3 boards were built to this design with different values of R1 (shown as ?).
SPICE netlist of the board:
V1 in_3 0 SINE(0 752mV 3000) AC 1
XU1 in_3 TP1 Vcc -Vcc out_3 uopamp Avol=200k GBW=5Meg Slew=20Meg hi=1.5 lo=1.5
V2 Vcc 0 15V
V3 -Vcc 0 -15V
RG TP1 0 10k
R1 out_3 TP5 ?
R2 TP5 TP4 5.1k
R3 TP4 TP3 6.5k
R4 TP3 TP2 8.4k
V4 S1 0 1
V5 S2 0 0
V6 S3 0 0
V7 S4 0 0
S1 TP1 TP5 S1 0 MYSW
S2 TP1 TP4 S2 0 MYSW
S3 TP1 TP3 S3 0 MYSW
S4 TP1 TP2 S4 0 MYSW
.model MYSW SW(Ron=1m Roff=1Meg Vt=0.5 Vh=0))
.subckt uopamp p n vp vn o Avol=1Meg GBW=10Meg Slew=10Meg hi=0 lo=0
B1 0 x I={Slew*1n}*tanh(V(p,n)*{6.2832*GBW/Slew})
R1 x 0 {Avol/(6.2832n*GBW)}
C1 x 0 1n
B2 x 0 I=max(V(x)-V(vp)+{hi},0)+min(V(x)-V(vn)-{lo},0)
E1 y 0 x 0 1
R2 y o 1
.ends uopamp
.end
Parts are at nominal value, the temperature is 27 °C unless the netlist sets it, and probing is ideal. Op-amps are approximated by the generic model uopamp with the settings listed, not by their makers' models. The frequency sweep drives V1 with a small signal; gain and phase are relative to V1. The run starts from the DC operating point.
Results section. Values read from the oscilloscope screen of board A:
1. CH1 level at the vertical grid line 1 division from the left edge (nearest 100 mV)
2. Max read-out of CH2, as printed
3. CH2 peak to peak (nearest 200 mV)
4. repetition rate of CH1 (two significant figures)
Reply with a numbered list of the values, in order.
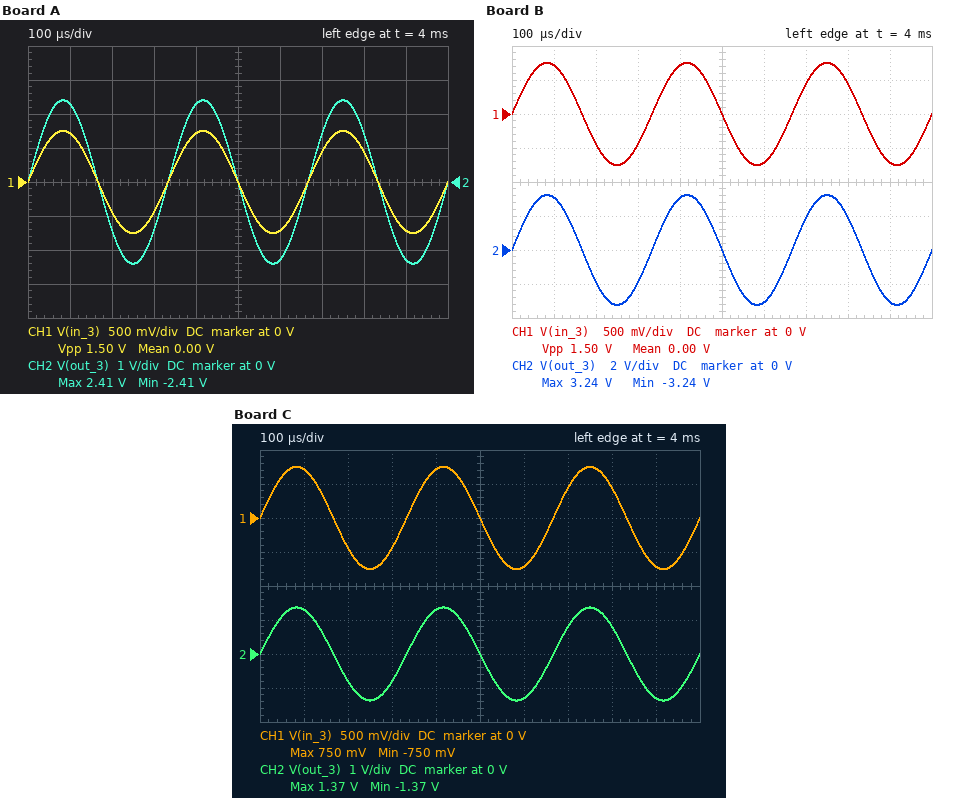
1. 700 mV
2. 2.41 V
3. 4.8 V
4. 3.0 kHz
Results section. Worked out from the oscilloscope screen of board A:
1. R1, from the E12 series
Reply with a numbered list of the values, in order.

1. 22 kΩ
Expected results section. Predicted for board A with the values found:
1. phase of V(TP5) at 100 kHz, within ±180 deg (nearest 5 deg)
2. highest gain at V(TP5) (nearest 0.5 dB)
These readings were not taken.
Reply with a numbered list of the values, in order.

1. -30 deg
2. 28.5 dB
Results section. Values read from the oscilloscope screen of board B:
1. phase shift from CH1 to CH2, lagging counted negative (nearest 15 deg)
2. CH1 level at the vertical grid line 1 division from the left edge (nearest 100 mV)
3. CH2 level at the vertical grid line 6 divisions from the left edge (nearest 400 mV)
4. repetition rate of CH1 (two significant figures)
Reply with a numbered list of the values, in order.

1. 0 deg
2. 700 mV
3. -3.2 V
4. 3.0 kHz
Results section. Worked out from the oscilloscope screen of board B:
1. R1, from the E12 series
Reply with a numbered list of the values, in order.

1. 33 kΩ
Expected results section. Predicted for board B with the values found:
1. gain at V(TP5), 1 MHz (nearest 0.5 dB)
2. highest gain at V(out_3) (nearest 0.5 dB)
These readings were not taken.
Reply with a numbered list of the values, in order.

1. 13.0 dB
2. 29.5 dB
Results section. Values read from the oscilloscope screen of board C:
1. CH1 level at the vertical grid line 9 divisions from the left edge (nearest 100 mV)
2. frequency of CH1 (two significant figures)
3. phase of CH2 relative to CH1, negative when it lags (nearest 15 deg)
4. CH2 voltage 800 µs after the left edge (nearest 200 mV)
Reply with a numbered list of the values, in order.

1. -700 mV
2. 3.0 kHz
3. 0 deg
4. 800 mV
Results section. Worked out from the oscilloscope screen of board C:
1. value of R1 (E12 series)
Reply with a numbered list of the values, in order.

1. 8.2 kΩ
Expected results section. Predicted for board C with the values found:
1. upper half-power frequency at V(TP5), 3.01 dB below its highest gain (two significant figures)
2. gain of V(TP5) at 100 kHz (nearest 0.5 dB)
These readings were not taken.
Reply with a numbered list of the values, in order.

1. 180 kHz
2. 27.5 dB
